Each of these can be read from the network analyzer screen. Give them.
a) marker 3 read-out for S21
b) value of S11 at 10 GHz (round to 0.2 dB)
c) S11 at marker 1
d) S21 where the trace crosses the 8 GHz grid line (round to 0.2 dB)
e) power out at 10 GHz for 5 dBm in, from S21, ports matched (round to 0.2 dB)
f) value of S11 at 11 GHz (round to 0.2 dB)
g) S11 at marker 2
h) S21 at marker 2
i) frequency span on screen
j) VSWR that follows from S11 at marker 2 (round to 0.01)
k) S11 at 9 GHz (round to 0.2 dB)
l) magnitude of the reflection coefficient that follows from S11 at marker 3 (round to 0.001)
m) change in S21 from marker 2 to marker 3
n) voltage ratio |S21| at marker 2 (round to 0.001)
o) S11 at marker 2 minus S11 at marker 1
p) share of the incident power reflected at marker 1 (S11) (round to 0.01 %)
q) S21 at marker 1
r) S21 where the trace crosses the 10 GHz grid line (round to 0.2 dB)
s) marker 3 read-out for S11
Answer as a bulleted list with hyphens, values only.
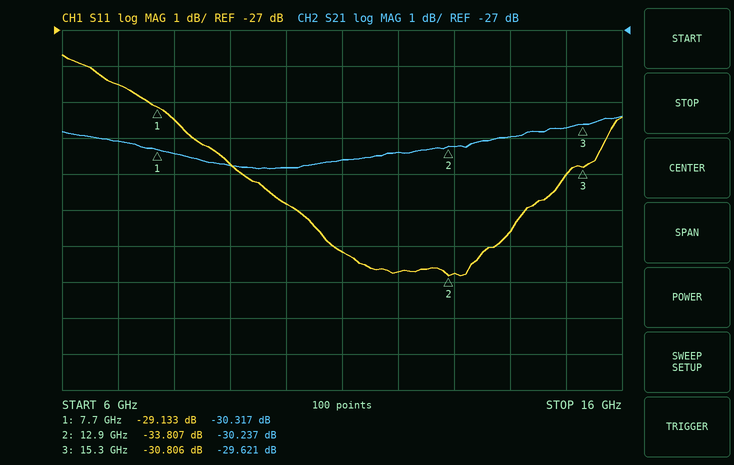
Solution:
- -29.621 dB
- -31.8 dB
- -29.133 dB
- -30.4 dB
- -25.8 dBm
- -33.2 dB
- -33.807 dB
- -30.237 dB
- 10 GHz
- 1.04
- -30.8 dB
- 0.029
- 0.616 dB
- 0.031
- -4.674 dB
- 0.12 %
- -30.317 dB
- -30.8 dB
- -30.806 dB
